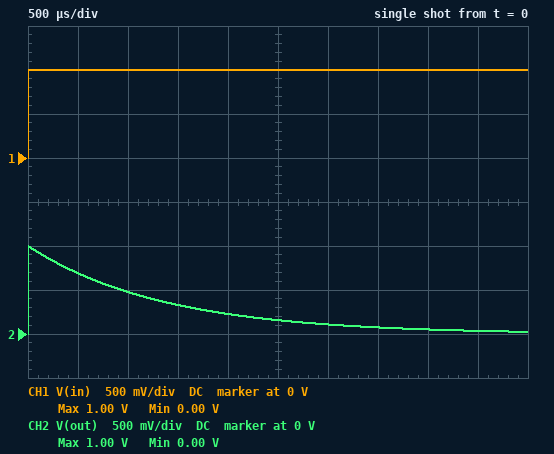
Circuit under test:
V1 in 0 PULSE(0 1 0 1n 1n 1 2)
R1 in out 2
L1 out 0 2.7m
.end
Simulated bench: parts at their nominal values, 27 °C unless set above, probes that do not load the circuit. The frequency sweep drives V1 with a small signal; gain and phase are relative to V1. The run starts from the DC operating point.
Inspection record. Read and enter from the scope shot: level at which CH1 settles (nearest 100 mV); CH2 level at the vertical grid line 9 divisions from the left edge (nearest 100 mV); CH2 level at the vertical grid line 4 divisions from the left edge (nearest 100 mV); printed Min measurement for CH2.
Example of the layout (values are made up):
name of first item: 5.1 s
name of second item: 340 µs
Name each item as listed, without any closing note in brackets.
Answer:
level at which CH1 settles: 1.0 V
CH2 level at the vertical grid line 9 divisions from the left edge: 0 V
CH2 level at the vertical grid line 4 divisions from the left edge: 200 mV
printed Min measurement for CH2: 0.00 V
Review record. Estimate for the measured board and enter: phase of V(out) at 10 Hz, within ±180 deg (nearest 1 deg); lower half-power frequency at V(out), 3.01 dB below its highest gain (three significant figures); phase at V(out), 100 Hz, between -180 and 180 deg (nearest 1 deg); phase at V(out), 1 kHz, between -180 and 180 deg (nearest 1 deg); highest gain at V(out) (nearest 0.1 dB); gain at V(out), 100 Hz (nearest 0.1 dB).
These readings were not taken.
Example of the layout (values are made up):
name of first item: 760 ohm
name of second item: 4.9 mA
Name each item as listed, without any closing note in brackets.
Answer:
phase of V(out) at 10 Hz, within ±180 deg: 85 deg
lower half-power frequency at V(out), 3.01 dB below its highest gain: 118 Hz
phase at V(out), 100 Hz, between -180 and 180 deg: 50 deg
phase at V(out), 1 kHz, between -180 and 180 deg: 7 deg
highest gain at V(out): 0 dB
gain at V(out), 100 Hz: -3.8 dB
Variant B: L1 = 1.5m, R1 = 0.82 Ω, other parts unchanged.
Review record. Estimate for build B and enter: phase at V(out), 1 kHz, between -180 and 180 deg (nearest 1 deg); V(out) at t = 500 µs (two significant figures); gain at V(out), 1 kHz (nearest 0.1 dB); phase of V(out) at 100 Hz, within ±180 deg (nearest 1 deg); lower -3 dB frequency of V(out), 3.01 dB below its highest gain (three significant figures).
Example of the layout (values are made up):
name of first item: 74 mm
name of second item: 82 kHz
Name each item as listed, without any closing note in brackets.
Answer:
phase at V(out), 1 kHz, between -180 and 180 deg: 5 deg
V(out) at t = 500 µs: 760 mV
gain at V(out), 1 kHz: 0 dB
phase of V(out) at 100 Hz, within ±180 deg: 41 deg
lower -3 dB frequency of V(out), 3.01 dB below its highest gain: 87.0 Hz
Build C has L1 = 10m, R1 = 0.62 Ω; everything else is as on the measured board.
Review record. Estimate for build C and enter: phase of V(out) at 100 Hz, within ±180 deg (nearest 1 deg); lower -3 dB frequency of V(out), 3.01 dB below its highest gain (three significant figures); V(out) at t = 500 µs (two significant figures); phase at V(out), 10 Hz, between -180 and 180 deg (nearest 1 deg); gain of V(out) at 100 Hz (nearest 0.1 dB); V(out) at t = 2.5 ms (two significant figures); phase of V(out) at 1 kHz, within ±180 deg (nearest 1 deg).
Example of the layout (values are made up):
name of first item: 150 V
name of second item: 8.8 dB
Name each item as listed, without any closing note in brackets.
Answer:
phase of V(out) at 100 Hz, within ±180 deg: 6 deg
lower -3 dB frequency of V(out), 3.01 dB below its highest gain: 9.87 Hz
V(out) at t = 500 µs: 970 mV
phase at V(out), 10 Hz, between -180 and 180 deg: 45 deg
gain of V(out) at 100 Hz: 0 dB
V(out) at t = 2.5 ms: 860 mV
phase of V(out) at 1 kHz, within ±180 deg: 1 deg
